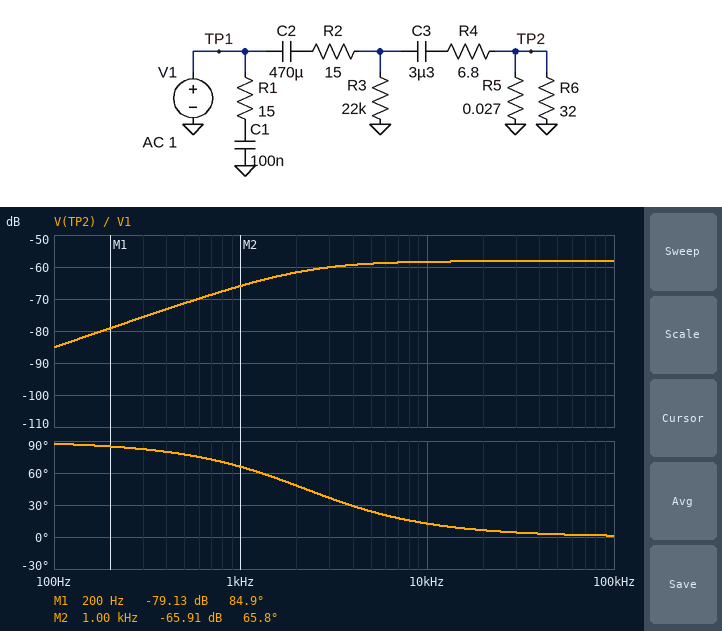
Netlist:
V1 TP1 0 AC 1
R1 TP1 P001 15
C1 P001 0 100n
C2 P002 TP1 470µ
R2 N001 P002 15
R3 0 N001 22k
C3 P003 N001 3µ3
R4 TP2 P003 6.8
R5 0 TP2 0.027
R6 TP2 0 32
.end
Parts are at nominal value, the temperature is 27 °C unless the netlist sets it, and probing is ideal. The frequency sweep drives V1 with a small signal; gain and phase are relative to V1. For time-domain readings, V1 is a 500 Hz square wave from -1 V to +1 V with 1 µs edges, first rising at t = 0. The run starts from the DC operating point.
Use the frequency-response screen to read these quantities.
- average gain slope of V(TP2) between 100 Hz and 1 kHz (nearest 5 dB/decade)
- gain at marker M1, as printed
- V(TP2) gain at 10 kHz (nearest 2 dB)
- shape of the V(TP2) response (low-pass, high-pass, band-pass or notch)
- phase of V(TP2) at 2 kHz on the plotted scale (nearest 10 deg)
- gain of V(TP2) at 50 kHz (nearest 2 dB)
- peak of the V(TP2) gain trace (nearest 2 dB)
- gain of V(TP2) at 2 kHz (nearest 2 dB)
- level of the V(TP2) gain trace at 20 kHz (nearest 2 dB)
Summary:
20 dB/decade
-79.13 dB
-58 dB
high-pass
50 deg
-58 dB
-58 dB
-62 dB
-58 dB
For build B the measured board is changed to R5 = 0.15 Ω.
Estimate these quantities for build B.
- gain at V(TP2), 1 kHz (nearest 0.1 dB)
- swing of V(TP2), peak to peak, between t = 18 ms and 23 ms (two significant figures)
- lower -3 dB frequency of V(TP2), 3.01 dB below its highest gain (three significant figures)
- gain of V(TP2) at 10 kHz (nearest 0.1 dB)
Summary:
-51.1 dB
27 mV
2.21 kHz
-43.6 dB
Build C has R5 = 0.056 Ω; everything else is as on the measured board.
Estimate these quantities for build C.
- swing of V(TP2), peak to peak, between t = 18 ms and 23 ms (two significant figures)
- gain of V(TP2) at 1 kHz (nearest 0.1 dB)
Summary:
10 mV
-59.6 dB
